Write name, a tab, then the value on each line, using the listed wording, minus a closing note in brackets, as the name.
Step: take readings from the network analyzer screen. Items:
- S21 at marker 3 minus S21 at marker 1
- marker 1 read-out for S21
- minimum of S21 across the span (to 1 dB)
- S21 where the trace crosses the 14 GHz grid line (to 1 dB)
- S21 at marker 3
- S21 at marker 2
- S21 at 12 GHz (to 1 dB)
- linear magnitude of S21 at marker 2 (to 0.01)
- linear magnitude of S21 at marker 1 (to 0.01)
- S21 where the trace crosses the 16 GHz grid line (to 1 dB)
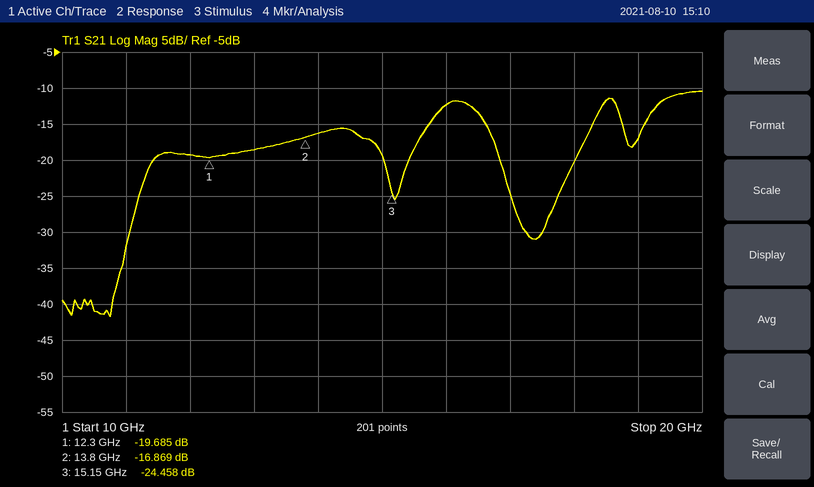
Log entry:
S21 at marker 3 minus S21 at marker 1	-4.773 dB
marker 1 read-out for S21	-19.685 dB
minimum of S21 across the span	-42 dB
S21 where the trace crosses the 14 GHz grid line	-16 dB
S21 at marker 3	-24.458 dB
S21 at marker 2	-16.869 dB
S21 at 12 GHz	-19 dB
linear magnitude of S21 at marker 2	0.14
linear magnitude of S21 at marker 1	0.10
S21 where the trace crosses the 16 GHz grid line	-12 dB
